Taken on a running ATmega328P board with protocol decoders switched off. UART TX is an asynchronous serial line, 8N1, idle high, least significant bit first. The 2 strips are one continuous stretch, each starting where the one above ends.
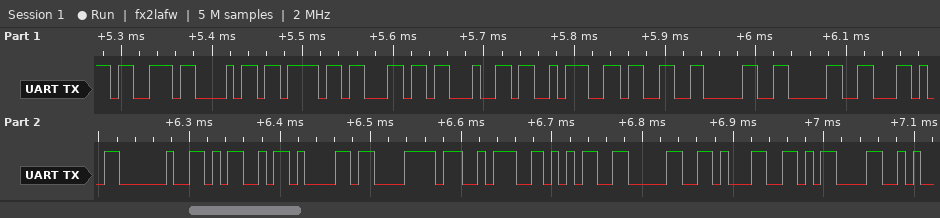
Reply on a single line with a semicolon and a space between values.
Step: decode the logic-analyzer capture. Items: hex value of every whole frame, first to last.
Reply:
73 68 6F 6C 64 3A 33 30 30 2C 20 4D 61 78 3A 35 30 31 0D
